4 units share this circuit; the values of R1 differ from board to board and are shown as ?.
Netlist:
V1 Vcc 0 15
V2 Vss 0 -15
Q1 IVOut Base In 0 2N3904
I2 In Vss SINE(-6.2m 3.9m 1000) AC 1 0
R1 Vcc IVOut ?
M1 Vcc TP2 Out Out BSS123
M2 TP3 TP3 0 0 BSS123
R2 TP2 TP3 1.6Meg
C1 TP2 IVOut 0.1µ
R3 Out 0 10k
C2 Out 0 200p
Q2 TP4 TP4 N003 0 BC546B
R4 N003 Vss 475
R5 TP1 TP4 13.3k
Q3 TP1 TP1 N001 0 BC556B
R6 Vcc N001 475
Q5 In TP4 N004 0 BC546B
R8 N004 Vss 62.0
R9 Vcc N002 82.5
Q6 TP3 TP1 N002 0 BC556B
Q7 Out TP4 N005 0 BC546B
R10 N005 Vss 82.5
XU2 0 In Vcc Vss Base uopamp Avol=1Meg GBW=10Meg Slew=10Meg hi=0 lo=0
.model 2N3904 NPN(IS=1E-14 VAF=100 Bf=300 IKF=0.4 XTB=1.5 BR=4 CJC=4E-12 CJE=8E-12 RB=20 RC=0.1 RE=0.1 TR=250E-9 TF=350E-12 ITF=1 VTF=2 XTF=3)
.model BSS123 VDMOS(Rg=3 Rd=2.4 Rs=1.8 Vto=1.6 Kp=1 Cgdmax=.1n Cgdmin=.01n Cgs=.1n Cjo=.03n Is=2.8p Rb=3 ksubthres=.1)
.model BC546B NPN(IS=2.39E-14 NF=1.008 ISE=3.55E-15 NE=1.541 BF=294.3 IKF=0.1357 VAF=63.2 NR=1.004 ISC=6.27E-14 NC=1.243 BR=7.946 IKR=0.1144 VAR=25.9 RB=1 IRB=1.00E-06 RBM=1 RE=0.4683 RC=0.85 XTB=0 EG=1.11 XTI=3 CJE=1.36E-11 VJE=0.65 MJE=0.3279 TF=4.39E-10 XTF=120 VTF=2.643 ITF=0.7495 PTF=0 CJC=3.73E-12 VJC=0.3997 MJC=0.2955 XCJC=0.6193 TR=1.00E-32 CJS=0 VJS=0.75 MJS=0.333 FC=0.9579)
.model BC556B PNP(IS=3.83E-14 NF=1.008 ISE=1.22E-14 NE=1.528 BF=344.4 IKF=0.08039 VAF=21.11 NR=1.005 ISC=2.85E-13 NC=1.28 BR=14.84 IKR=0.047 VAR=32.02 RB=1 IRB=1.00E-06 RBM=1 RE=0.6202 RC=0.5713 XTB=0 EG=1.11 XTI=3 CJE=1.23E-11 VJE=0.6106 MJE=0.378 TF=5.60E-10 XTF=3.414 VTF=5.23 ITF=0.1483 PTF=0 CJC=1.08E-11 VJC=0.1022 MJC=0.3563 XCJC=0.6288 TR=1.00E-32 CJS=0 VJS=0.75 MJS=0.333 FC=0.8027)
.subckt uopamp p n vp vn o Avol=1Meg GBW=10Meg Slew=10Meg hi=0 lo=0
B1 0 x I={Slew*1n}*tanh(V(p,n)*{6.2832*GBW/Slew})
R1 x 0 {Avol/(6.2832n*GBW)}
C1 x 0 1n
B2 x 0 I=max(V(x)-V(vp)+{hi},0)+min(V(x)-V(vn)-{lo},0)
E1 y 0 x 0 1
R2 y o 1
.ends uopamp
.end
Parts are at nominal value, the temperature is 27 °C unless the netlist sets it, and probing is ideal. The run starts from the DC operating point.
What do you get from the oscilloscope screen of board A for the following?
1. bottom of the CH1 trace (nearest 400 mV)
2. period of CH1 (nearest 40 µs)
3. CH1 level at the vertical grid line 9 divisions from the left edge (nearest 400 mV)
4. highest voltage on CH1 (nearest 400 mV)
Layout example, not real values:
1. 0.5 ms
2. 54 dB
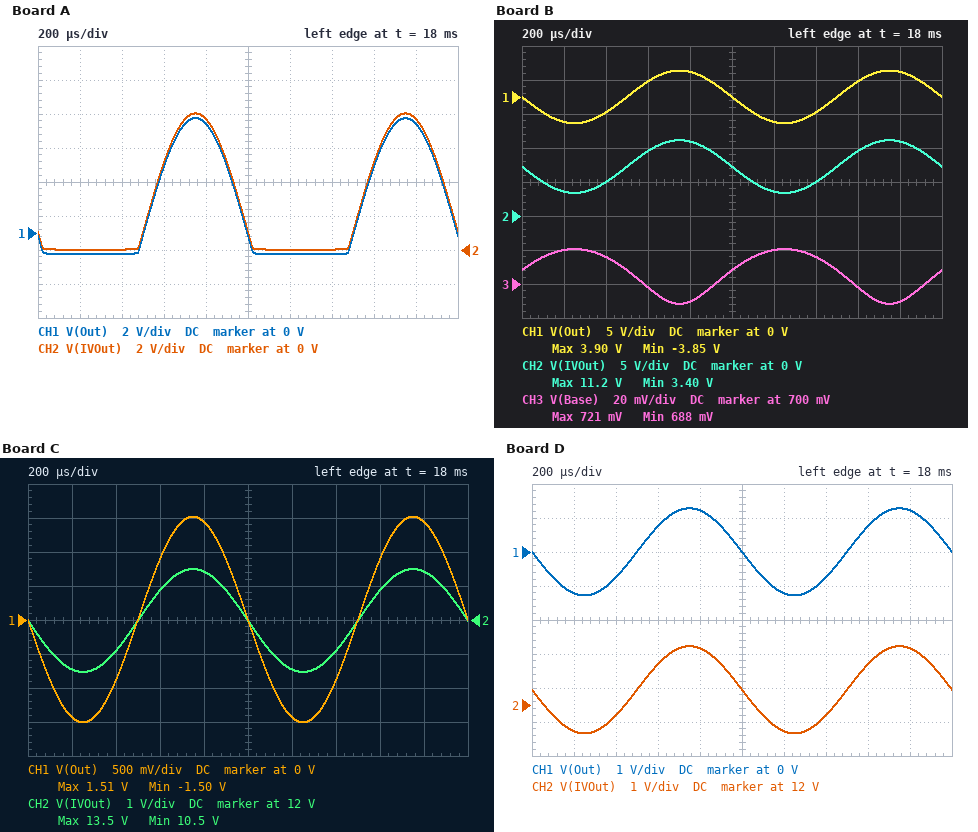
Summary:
1. -1.2 V
2. 1.00 ms
3. 6.4 V
4. 6.8 V
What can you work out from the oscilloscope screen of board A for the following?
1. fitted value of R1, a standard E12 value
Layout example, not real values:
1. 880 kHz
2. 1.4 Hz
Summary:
1. 1.8 kΩ
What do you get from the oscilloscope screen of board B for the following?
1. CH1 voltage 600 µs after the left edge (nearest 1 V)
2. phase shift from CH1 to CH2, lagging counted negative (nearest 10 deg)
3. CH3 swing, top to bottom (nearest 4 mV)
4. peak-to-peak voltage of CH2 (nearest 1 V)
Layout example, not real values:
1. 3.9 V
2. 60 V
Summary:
1. 2 V
2. 0 deg
3. 32 mV
4. 8 V
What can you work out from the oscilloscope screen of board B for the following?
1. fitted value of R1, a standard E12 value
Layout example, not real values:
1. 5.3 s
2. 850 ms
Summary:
1. 1 kΩ
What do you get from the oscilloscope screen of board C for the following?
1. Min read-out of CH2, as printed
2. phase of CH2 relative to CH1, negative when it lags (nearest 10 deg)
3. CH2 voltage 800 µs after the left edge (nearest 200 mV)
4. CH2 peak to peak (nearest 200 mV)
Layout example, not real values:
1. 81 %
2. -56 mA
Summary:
1. 10.5 V
2. 0 deg
3. 13.4 V
4. 3.0 V
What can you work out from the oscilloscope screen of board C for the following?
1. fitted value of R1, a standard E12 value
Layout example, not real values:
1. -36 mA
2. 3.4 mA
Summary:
1. 390 Ω
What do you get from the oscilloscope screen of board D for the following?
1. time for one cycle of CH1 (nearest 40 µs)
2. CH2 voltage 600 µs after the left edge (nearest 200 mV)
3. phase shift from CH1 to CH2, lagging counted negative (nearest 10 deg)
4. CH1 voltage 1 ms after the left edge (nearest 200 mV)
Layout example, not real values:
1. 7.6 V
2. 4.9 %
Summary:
1. 1.00 ms
2. 13.2 V
3. 0 deg
4. 0 V
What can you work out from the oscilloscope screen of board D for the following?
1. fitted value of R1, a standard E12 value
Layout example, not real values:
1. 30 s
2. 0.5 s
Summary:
1. 330 Ω
